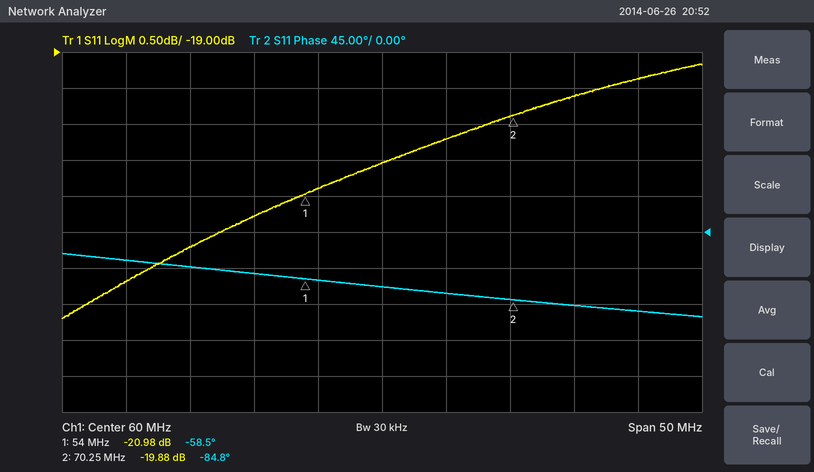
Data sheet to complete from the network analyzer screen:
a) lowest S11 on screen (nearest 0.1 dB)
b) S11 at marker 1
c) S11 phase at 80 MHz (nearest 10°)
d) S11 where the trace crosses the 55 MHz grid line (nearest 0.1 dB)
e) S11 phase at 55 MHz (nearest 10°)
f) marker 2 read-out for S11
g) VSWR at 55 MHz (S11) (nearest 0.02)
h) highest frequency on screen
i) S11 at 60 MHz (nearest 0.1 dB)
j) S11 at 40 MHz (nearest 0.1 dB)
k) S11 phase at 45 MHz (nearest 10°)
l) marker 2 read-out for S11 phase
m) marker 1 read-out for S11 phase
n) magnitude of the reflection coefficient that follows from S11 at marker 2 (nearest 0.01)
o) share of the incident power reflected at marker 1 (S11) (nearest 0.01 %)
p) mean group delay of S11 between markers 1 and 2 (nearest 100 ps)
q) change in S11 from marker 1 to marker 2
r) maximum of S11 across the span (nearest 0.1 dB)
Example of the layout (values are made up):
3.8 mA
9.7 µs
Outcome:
-22.7 dB
-20.98 dB
-100°
-20.9 dB
-60°
-19.88 dB
1.20
85 MHz
-20.5 dB
-22.2 dB
-40°
-84.8°
-58.5°
0.10
0.80 %
4.5 ns
1.10 dB
-19.2 dB
